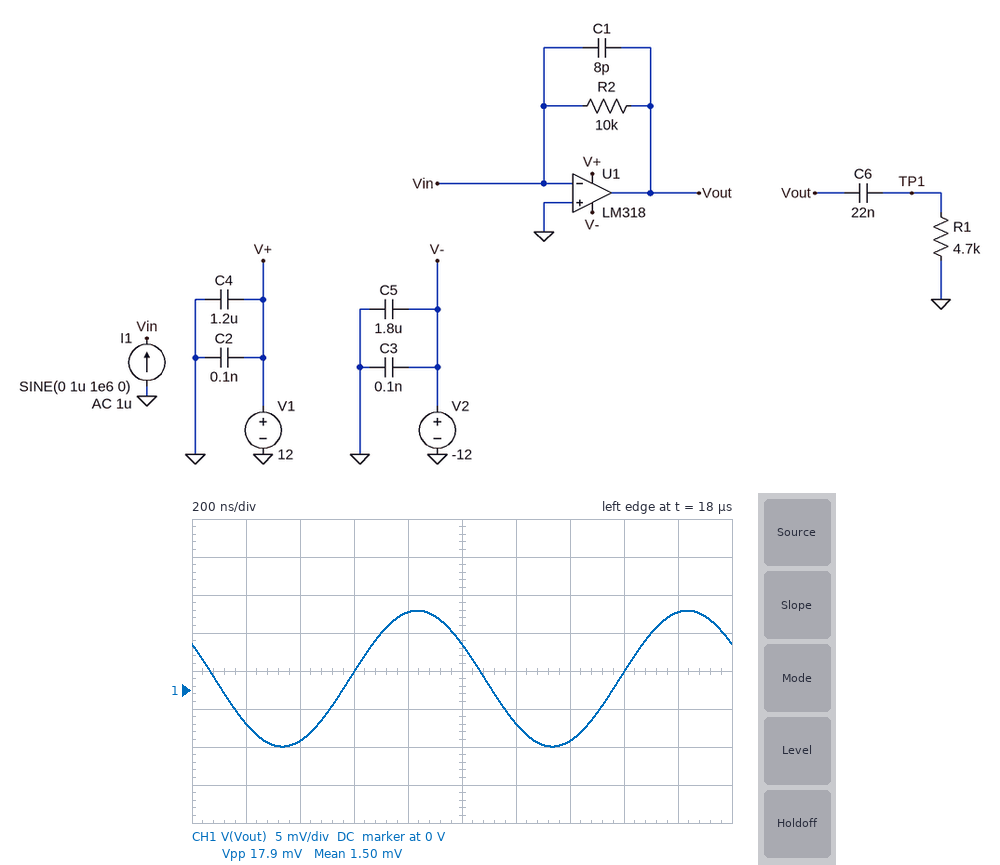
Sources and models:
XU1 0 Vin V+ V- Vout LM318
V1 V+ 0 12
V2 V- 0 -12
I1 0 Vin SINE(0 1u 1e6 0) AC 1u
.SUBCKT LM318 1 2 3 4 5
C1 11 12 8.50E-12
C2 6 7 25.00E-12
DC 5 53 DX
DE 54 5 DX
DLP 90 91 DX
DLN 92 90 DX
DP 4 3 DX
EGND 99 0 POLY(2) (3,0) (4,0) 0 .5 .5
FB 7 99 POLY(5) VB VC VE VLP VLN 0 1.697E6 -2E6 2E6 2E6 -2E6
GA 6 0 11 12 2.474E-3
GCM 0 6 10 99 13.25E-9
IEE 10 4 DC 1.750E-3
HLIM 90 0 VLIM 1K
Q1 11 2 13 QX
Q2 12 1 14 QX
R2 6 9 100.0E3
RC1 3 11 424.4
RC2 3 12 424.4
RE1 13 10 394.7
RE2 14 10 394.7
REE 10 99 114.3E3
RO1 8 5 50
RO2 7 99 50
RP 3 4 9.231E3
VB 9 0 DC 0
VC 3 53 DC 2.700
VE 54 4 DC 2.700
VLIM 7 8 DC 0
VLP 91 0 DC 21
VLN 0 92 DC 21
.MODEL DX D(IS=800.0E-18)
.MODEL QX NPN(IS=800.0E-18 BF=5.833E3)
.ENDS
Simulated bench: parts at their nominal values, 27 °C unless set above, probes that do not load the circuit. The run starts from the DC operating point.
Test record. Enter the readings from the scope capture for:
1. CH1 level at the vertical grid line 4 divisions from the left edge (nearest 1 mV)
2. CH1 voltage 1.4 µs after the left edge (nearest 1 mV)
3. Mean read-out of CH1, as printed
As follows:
10 mV
-7 mV
1.50 mV
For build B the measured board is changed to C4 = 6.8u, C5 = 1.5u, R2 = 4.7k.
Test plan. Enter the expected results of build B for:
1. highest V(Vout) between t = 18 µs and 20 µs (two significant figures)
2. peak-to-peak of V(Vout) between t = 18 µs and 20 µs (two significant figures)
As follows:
5.3 mV
9.2 mV
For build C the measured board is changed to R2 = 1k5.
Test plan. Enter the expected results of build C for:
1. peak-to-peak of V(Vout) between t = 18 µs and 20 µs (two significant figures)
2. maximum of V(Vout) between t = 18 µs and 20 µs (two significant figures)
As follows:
3.0 mV
1.7 mV
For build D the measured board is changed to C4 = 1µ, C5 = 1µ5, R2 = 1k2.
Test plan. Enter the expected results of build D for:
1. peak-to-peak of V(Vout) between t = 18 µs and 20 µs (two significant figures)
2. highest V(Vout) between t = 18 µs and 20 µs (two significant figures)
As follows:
2.4 mV
1.4 mV
